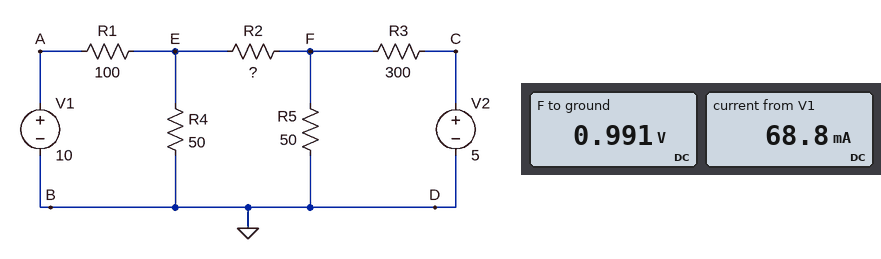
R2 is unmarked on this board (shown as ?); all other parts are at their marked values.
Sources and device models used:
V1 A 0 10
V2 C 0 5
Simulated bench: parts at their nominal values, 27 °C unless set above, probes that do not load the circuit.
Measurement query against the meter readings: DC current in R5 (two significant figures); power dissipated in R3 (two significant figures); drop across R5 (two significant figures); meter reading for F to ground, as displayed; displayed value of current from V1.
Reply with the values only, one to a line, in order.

20 mA
54 mW
990 mV
0.991 V
68.8 mA
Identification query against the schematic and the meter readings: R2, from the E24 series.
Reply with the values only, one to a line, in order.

330 Ω
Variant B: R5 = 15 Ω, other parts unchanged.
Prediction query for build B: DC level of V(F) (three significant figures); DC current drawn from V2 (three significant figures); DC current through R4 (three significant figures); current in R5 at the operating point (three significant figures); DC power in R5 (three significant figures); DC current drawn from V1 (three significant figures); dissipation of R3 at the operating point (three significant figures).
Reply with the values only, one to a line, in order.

355 mV
15.5 mA
61.2 mA
23.7 mA
8.41 mW
69.4 mA
71.9 mW
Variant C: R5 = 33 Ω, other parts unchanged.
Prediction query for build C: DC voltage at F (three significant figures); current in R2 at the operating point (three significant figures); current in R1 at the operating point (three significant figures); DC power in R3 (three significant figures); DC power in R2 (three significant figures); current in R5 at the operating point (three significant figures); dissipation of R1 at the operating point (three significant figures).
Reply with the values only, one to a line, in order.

710 mV
7.22 mA
69.1 mA
61.3 mW
17.2 mW
21.5 mA
477 mW
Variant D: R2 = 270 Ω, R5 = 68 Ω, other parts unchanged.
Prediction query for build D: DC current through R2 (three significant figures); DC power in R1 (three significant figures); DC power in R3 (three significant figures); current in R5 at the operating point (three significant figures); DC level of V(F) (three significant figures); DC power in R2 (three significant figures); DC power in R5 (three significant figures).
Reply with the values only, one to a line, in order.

6.72 mA
475 mW
45.7 mW
19.1 mA
1.30 V
12.2 mW
24.7 mW
